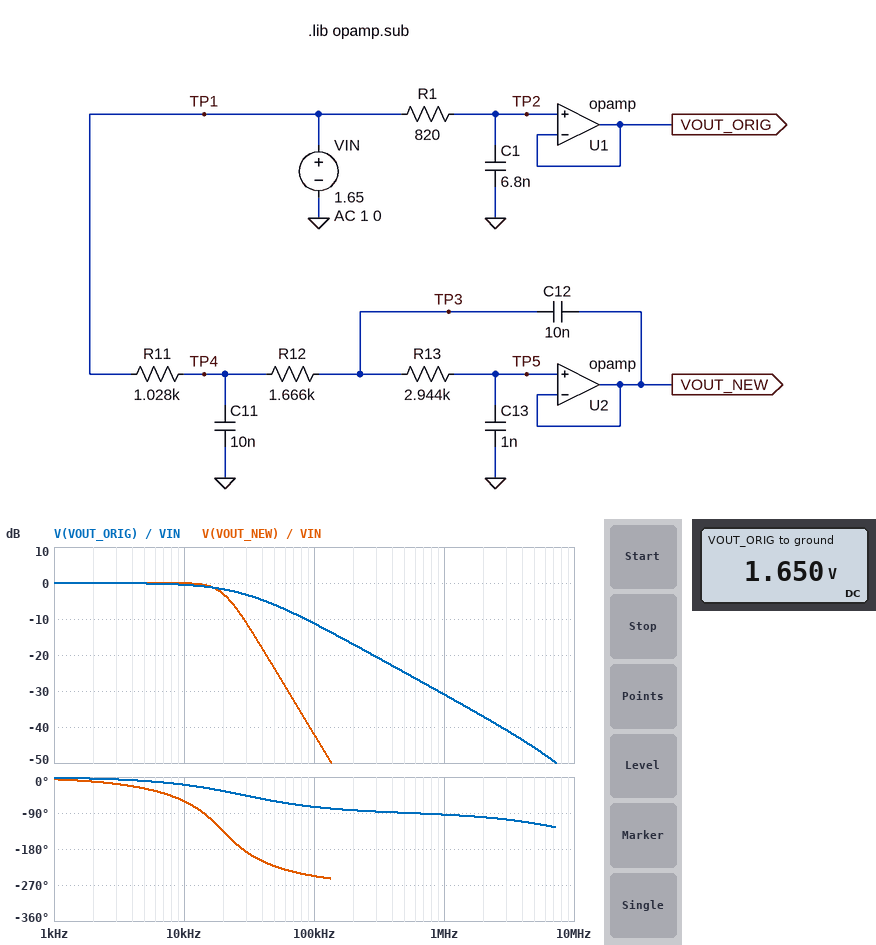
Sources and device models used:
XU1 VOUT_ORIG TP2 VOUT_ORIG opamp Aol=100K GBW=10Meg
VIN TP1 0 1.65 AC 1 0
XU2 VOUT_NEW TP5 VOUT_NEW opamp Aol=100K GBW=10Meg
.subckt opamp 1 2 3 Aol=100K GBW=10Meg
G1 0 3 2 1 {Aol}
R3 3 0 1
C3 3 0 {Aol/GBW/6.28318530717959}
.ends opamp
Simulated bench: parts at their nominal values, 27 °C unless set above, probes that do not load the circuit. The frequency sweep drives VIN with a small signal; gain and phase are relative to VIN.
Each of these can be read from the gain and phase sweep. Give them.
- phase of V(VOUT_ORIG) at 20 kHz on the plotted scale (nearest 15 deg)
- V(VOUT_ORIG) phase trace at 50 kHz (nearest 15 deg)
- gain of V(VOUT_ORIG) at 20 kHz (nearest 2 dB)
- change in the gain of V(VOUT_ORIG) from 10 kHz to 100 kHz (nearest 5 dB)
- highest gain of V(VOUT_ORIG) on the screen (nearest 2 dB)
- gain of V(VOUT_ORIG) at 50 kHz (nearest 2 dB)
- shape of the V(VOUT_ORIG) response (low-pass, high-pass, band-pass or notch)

-30 deg
-60 deg
-2 dB
-10 dB
0 dB
-6 dB
low-pass
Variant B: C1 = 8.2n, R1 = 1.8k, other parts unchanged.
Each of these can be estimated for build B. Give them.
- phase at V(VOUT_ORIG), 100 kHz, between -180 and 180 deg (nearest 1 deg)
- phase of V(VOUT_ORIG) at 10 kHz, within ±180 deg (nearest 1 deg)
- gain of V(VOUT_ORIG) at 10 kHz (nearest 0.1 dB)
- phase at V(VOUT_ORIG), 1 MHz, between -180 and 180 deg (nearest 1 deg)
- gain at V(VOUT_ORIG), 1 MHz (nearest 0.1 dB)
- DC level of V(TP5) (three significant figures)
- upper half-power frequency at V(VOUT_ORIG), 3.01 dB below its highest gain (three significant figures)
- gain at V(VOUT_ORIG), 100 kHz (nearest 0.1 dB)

-84 deg
-43 deg
-2.7 dB
-95 deg
-39.4 dB
1.65 V
10.8 kHz
-19.4 dB
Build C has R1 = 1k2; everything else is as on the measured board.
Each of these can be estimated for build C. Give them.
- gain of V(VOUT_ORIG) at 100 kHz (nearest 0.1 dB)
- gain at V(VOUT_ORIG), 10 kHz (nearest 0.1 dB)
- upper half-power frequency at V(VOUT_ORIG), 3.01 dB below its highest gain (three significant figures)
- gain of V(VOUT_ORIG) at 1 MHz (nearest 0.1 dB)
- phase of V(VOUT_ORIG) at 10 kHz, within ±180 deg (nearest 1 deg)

-14.4 dB
-1.0 dB
19.5 kHz
-34.2 dB
-27 deg
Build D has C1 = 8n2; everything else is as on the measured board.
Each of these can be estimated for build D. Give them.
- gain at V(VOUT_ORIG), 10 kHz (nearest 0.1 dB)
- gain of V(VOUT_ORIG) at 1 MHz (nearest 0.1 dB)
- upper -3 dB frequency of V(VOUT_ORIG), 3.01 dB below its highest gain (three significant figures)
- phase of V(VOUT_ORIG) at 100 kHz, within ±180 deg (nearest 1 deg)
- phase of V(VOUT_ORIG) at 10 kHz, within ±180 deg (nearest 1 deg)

-0.7 dB
-32.6 dB
23.7 kHz
-77 deg
-23 deg
